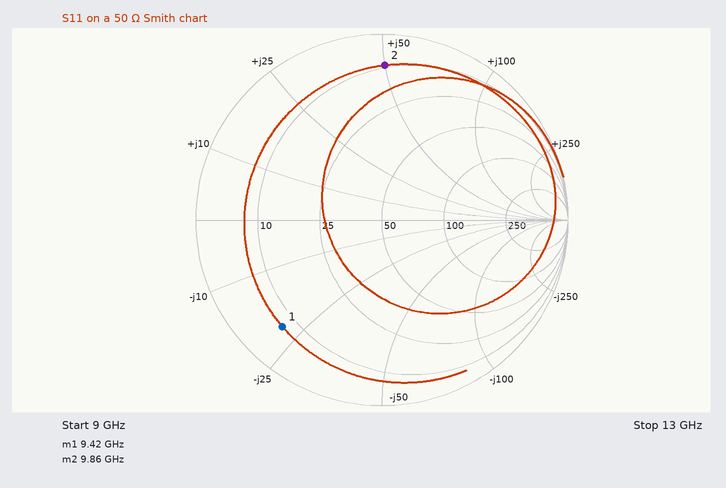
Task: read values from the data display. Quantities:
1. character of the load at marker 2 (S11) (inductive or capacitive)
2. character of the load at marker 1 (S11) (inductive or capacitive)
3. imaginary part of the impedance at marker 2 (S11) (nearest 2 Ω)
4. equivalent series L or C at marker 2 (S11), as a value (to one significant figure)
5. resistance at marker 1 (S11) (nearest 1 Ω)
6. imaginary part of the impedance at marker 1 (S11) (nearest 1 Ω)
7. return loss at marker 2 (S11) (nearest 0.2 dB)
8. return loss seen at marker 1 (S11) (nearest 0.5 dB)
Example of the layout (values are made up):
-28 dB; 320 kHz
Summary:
inductive; capacitive; +50 Ω; 800 pH; 7 Ω; -21 Ω; 1.6 dB; 2.0 dB
